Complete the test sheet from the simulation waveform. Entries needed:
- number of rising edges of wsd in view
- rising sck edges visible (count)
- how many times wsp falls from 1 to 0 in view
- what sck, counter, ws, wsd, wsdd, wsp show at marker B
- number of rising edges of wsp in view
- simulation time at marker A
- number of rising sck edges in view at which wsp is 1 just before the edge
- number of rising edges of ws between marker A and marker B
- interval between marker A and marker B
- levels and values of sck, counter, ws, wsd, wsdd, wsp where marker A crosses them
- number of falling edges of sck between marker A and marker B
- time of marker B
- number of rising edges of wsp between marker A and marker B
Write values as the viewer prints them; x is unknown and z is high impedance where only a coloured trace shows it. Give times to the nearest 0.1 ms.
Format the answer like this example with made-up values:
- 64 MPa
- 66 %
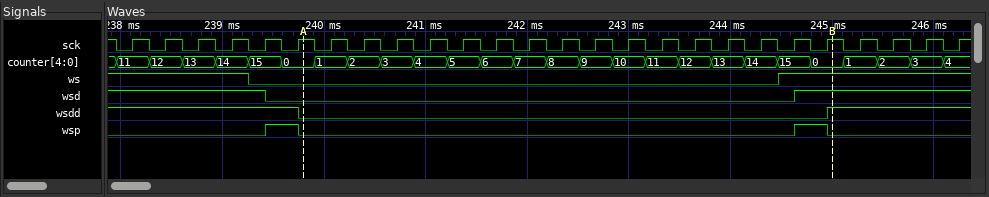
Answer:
- 1
- 26
- 2
- sck=1, counter=0, ws=1, wsd=1, wsdd=1, wsp=0
- 2
- 239.8 ms
- 2
- 1
- 5.2 ms
- sck=1, counter=0, ws=0, wsd=0, wsdd=0, wsp=0
- 16
- 245 ms
- 1
